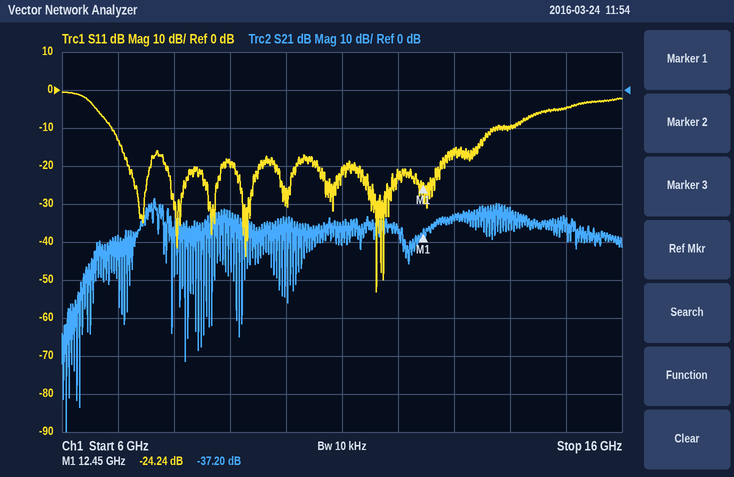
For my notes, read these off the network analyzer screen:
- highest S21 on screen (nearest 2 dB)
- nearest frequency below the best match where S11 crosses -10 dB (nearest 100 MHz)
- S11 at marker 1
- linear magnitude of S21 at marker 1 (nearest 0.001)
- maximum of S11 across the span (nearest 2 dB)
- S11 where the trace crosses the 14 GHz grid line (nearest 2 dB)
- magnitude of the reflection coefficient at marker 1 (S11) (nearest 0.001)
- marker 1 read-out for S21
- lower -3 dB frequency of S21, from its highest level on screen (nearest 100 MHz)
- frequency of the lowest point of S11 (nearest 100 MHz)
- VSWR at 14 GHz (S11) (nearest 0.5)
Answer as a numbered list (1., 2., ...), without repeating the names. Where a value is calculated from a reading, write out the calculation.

1. -28 dB
2. 6.9 GHz
3. -24.24 dB
4. 10^(-37.2/20) ≈ 0.014
5. 0 dB
6. -10 dB
7. 10^(-24.24/20) ≈ 0.061
8. -37.20 dB
9. 7.6 GHz
10. 11.6 GHz
11. |Γ| = 10^(-10/20) = 0.3162; VSWR = (1 + 0.3162)/(1 − 0.3162) ≈ 1.92, so 2.0 to the nearest 0.5
